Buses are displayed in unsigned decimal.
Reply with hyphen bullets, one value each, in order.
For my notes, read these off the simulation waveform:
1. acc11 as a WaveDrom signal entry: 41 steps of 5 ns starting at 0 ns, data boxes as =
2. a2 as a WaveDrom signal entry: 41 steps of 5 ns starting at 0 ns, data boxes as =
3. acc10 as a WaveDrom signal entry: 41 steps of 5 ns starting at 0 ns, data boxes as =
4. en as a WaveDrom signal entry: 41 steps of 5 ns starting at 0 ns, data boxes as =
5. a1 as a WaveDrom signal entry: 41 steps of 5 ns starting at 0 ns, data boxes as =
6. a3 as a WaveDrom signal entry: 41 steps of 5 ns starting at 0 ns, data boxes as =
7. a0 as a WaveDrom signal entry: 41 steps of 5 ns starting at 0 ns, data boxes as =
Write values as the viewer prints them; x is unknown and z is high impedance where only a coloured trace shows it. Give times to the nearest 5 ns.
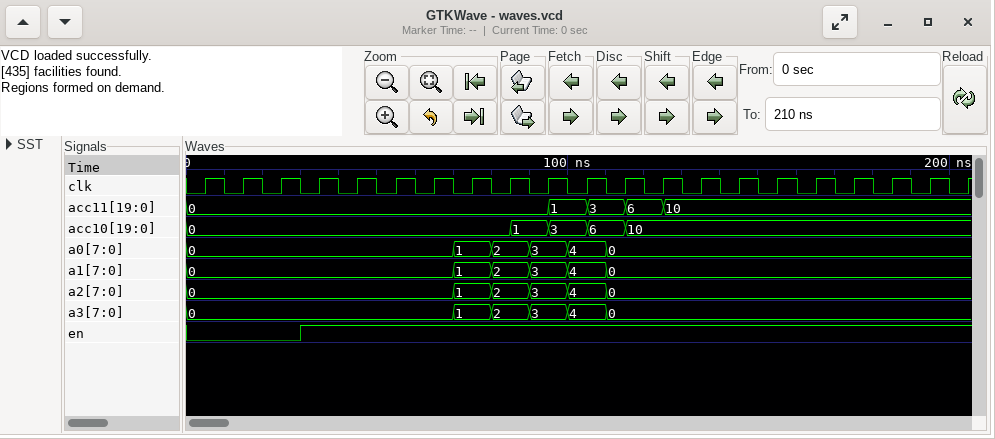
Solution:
- {name: 'acc11', wave: '=..................=.=.=.=...............', data: '0 1 3 6 10'}
- {name: 'a2', wave: '=.............=.=.=.=.=..................', data: '0 1 2 3 4 0'}
- {name: 'acc10', wave: '=................=.=.=.=.................', data: '0 1 3 6 10'}
- {name: 'en', wave: '0.....1..................................'}
- {name: 'a1', wave: '=.............=.=.=.=.=..................', data: '0 1 2 3 4 0'}
- {name: 'a3', wave: '=.............=.=.=.=.=..................', data: '0 1 2 3 4 0'}
- {name: 'a0', wave: '=.............=.=.=.=.=..................', data: '0 1 2 3 4 0'}
